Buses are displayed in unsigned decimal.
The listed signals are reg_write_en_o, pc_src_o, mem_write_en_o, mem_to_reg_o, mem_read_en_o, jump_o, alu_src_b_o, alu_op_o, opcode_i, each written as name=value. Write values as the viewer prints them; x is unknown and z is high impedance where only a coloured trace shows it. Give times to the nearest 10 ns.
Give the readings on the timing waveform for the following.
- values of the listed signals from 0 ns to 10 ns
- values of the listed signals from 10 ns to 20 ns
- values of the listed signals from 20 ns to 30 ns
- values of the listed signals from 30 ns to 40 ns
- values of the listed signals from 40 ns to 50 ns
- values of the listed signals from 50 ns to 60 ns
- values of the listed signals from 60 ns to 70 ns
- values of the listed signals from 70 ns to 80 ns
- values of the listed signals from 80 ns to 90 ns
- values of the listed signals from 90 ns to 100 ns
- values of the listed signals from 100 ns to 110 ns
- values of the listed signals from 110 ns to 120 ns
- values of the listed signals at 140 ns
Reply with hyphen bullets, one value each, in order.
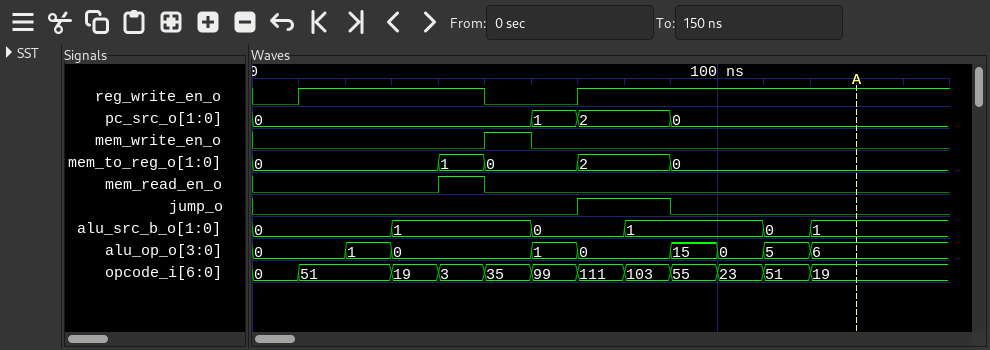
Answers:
- reg_write_en_o=0, pc_src_o=0, mem_write_en_o=0, mem_to_reg_o=0, mem_read_en_o=0, jump_o=0, alu_src_b_o=0, alu_op_o=0, opcode_i=0
- reg_write_en_o=1, pc_src_o=0, mem_write_en_o=0, mem_to_reg_o=0, mem_read_en_o=0, jump_o=0, alu_src_b_o=0, alu_op_o=0, opcode_i=51
- reg_write_en_o=1, pc_src_o=0, mem_write_en_o=0, mem_to_reg_o=0, mem_read_en_o=0, jump_o=0, alu_src_b_o=0, alu_op_o=1, opcode_i=51
- reg_write_en_o=1, pc_src_o=0, mem_write_en_o=0, mem_to_reg_o=0, mem_read_en_o=0, jump_o=0, alu_src_b_o=1, alu_op_o=0, opcode_i=19
- reg_write_en_o=1, pc_src_o=0, mem_write_en_o=0, mem_to_reg_o=1, mem_read_en_o=1, jump_o=0, alu_src_b_o=1, alu_op_o=0, opcode_i=3
- reg_write_en_o=0, pc_src_o=0, mem_write_en_o=1, mem_to_reg_o=0, mem_read_en_o=0, jump_o=0, alu_src_b_o=1, alu_op_o=0, opcode_i=35
- reg_write_en_o=0, pc_src_o=1, mem_write_en_o=0, mem_to_reg_o=0, mem_read_en_o=0, jump_o=0, alu_src_b_o=0, alu_op_o=1, opcode_i=99
- reg_write_en_o=1, pc_src_o=2, mem_write_en_o=0, mem_to_reg_o=2, mem_read_en_o=0, jump_o=1, alu_src_b_o=0, alu_op_o=0, opcode_i=111
- reg_write_en_o=1, pc_src_o=2, mem_write_en_o=0, mem_to_reg_o=2, mem_read_en_o=0, jump_o=1, alu_src_b_o=1, alu_op_o=0, opcode_i=103
- reg_write_en_o=1, pc_src_o=0, mem_write_en_o=0, mem_to_reg_o=0, mem_read_en_o=0, jump_o=0, alu_src_b_o=1, alu_op_o=15, opcode_i=55
- reg_write_en_o=1, pc_src_o=0, mem_write_en_o=0, mem_to_reg_o=0, mem_read_en_o=0, jump_o=0, alu_src_b_o=1, alu_op_o=0, opcode_i=23
- reg_write_en_o=1, pc_src_o=0, mem_write_en_o=0, mem_to_reg_o=0, mem_read_en_o=0, jump_o=0, alu_src_b_o=0, alu_op_o=5, opcode_i=51
- reg_write_en_o=1, pc_src_o=0, mem_write_en_o=0, mem_to_reg_o=0, mem_read_en_o=0, jump_o=0, alu_src_b_o=1, alu_op_o=6, opcode_i=19
